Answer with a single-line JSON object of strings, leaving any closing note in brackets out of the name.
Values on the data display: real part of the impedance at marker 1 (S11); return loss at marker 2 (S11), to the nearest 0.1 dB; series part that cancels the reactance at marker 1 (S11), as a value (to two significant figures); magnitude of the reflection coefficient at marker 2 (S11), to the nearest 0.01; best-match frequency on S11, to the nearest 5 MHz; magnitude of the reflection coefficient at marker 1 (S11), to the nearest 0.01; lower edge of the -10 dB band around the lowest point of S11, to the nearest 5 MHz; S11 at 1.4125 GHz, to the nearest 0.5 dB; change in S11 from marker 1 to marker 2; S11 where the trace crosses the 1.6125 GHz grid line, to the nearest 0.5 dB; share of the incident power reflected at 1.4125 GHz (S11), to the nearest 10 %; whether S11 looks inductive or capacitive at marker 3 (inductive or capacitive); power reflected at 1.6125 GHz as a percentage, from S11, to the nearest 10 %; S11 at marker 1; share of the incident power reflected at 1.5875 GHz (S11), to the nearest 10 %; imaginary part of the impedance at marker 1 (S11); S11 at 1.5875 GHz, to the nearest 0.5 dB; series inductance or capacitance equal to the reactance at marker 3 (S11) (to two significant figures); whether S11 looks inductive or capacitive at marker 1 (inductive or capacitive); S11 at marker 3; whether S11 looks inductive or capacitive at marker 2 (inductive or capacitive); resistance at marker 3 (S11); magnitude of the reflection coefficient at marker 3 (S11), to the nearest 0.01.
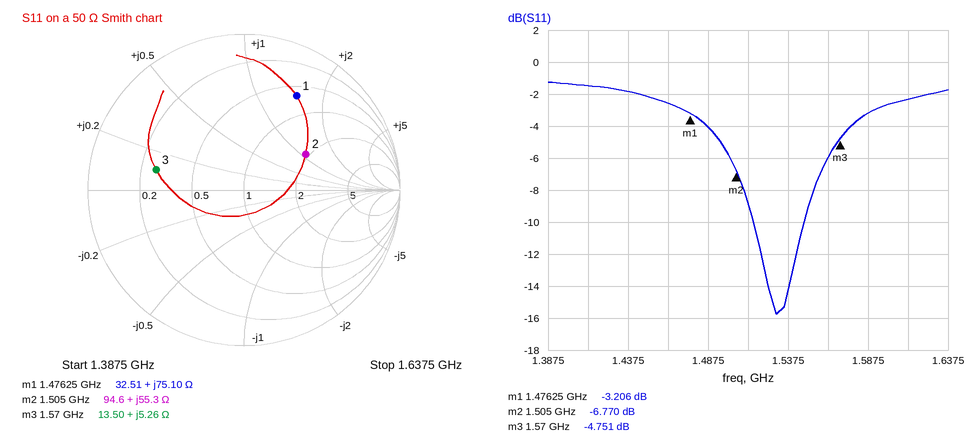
{"real part of the impedance at marker 1": "32.51 Ω", "return loss at marker 2 (S11), to the nearest 0.1 dB": "6.8 dB", "series part that cancels the reactance at marker 1 (S11), as a value": "1.4 pF", "magnitude of the reflection coefficient at marker 2 (S11), to the nearest 0.01": "0.46", "best-match frequency on S11, to the nearest 5 MHz": "1.530 GHz", "magnitude of the reflection coefficient at marker 1 (S11), to the nearest 0.01": "0.69", "lower edge of the -10 dB band around the lowest point of S11, to the nearest 5 MHz": "1.515 GHz", "S11 at 1.4125 GHz, to the nearest 0.5 dB": "-1.5 dB", "change in S11 from marker 1 to marker 2": "-3.564 dB", "S11 where the trace crosses the 1.6125 GHz grid line, to the nearest 0.5 dB": "-2.5 dB", "share of the incident power reflected at 1.4125 GHz (S11), to the nearest 10 %": "70 %", "whether S11 looks inductive or capacitive at marker 3": "inductive", "power reflected at 1.6125 GHz as a percentage, from S11, to the nearest 10 %": "60 %", "S11 at marker 1": "-3.206 dB", "share of the incident power reflected at 1.5875 GHz (S11), to the nearest 10 %": "50 %", "imaginary part of the impedance at marker 1": "+75.10 Ω", "S11 at 1.5875 GHz, to the nearest 0.5 dB": "-3.0 dB", "series inductance or capacitance equal to the reactance at marker 3 (S11)": "530 pH", "whether S11 looks inductive or capacitive at marker 1": "inductive", "S11 at marker 3": "-4.751 dB", "whether S11 looks inductive or capacitive at marker 2": "inductive", "resistance at marker 3": "13.50 Ω", "magnitude of the reflection coefficient at marker 3 (S11), to the nearest 0.01": "0.58"}
